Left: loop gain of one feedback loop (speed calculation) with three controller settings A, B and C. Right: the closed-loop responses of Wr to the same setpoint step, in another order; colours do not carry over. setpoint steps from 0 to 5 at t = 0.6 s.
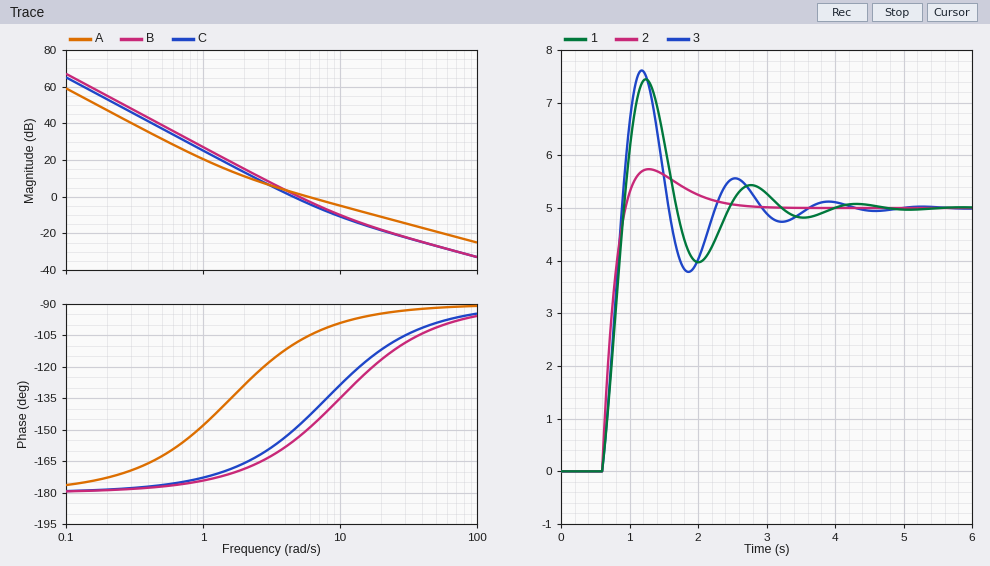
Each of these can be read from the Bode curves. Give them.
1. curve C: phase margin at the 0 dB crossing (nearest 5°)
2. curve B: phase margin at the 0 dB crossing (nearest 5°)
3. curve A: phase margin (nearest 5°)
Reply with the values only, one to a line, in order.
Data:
30°
25°
75°
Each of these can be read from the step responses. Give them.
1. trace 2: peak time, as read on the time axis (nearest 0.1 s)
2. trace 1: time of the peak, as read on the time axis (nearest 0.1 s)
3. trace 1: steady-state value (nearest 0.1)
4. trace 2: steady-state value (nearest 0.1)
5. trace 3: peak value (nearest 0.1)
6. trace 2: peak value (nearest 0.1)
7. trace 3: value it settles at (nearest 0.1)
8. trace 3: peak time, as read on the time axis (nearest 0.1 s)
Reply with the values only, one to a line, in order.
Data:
1.3 s
1.2 s
5.0
5.0
7.6
5.7
5.0
1.2 s
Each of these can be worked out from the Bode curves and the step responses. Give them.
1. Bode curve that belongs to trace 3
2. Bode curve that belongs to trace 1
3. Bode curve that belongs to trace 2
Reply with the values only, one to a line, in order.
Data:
B
C
A
